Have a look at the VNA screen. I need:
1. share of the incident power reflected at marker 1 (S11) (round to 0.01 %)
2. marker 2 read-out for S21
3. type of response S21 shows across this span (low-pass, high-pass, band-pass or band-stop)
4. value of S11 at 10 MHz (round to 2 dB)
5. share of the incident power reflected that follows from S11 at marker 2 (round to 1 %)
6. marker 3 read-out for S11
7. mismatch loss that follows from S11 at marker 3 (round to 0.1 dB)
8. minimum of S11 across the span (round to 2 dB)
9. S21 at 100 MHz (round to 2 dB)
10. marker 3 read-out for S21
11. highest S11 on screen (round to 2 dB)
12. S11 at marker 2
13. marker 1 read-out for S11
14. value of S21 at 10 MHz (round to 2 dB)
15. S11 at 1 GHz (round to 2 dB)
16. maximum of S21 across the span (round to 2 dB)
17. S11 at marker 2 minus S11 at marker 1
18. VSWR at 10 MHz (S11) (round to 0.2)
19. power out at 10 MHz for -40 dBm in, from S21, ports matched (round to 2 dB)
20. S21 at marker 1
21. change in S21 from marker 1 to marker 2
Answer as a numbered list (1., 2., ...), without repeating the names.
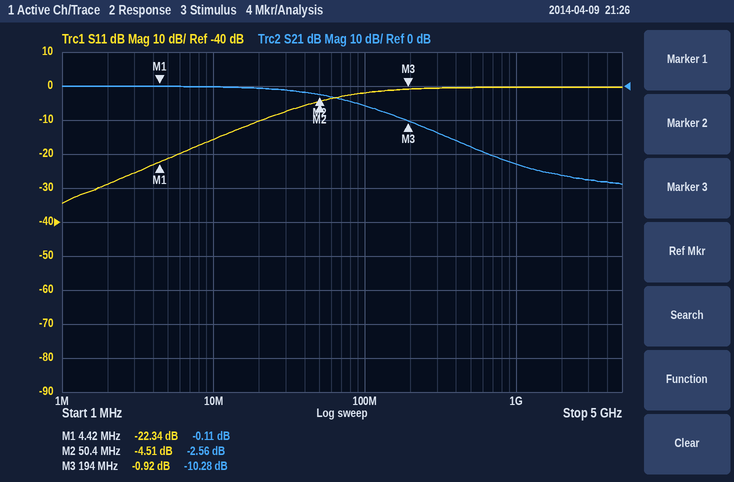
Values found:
1. 0.58 %
2. -2.56 dB
3. low-pass
4. -16 dB
5. 35 %
6. -0.92 dB
7. 7.2 dB
8. -34 dB
9. -6 dB
10. -10.28 dB
11. 0 dB
12. -4.51 dB
13. -22.34 dB
14. 0 dB
15. 0 dB
16. 0 dB
17. 17.83 dB
18. 1.4
19. -40 dBm
20. -0.11 dB
21. -2.45 dB
